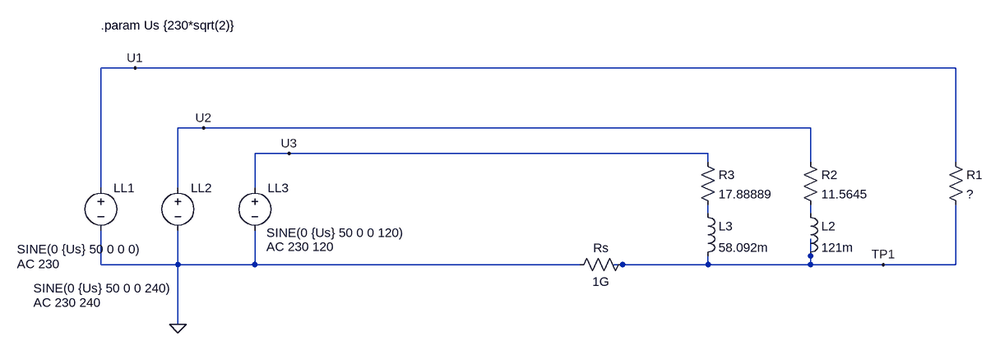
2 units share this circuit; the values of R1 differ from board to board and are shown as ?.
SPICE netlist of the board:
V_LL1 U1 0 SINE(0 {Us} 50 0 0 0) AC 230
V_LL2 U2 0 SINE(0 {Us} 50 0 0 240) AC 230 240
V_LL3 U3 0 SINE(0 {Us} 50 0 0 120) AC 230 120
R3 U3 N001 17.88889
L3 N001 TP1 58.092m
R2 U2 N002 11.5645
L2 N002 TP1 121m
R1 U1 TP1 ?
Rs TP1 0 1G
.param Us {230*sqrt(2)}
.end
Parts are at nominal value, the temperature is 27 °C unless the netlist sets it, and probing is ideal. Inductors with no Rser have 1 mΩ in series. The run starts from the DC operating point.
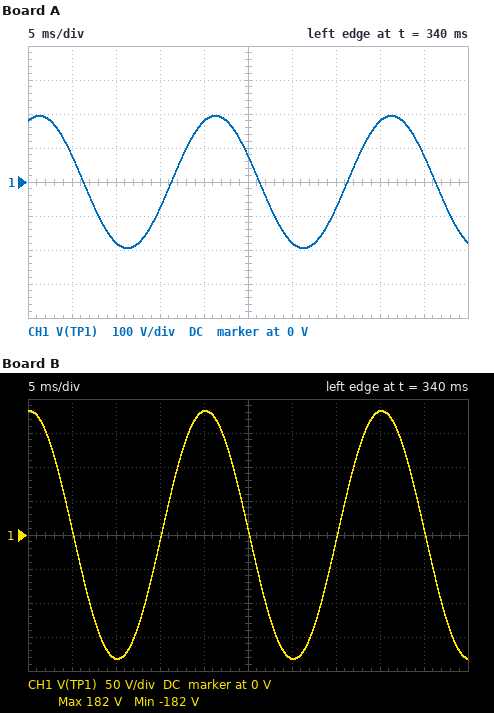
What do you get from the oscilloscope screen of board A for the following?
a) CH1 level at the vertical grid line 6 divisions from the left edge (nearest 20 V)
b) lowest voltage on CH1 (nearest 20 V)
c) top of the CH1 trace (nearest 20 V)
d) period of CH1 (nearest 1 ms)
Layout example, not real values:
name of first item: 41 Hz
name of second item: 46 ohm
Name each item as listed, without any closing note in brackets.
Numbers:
CH1 level at the vertical grid line 6 divisions from the left edge: -180 V
lowest voltage on CH1: -200 V
top of the CH1 trace: 200 V
period of CH1: 20 ms
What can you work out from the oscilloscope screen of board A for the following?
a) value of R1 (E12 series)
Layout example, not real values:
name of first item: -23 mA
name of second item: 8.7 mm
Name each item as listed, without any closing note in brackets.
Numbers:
value of R1: 15 Ω
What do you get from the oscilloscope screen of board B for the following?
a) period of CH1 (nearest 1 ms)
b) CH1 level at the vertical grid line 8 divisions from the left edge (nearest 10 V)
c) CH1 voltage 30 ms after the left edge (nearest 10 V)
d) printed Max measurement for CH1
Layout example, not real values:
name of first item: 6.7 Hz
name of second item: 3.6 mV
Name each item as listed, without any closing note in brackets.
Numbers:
period of CH1: 20 ms
CH1 level at the vertical grid line 8 divisions from the left edge: 180 V
CH1 voltage 30 ms after the left edge: -180 V
printed Max measurement for CH1: 182 V
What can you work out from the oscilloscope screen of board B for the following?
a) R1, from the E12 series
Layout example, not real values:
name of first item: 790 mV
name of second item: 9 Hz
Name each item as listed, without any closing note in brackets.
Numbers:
R1, from the E12 series: 22 Ω
